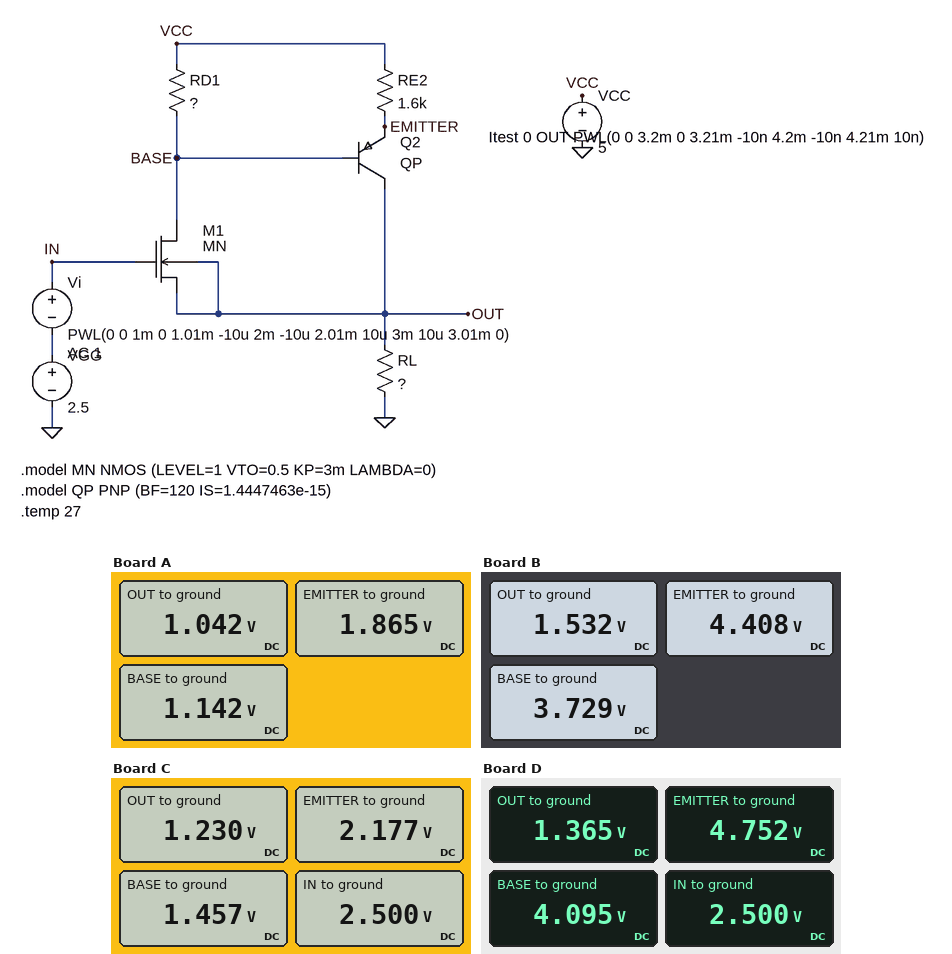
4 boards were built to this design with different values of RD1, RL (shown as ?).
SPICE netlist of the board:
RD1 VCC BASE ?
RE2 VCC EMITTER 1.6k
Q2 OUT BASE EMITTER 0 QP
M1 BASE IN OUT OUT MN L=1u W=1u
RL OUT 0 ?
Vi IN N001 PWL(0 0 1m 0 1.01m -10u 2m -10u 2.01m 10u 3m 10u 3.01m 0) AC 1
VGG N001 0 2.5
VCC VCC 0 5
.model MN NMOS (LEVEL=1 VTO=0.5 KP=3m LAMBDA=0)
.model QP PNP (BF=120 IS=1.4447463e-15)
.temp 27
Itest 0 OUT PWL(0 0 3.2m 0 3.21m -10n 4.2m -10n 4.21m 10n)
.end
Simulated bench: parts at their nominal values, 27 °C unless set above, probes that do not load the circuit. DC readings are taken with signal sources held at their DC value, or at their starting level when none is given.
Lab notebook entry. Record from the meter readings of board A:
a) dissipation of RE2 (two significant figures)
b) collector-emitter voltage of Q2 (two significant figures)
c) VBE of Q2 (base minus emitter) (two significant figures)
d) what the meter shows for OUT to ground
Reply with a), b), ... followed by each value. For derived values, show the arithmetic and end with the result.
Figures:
a) (5 V - 1.865 V)^2 / 1.6 kΩ = 6.1 mW
b) 1.042 V - 1.865 V = -820 mV
c) 1.142 V - 1.865 V = -720 mV
d) 1.042 V
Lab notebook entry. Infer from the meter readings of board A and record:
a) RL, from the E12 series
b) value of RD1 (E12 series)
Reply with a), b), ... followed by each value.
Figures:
a) 470 Ω
b) 15 kΩ
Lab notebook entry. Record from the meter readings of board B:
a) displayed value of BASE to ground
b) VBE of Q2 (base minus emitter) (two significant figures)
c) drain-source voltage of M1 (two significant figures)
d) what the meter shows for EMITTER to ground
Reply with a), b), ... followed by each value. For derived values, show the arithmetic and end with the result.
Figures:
a) 3.729 V
b) 3.729 V - 4.408 V = -680 mV
c) 3.729 V - 1.532 V = 2.2 V
d) 4.408 V
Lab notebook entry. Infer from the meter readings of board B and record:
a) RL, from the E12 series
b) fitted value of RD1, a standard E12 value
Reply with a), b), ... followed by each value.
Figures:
a) 2.2 kΩ
b) 3.9 kΩ
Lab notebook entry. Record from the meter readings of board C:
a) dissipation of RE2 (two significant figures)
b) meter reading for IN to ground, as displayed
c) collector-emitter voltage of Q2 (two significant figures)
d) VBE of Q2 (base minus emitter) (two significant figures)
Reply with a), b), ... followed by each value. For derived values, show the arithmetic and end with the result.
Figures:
a) (5 V - 2.177 V)^2 / 1.6 kΩ = 5.0 mW
b) 2.500 V
c) 1.23 V - 2.177 V = -950 mV
d) 1.457 V - 2.177 V = -720 mV
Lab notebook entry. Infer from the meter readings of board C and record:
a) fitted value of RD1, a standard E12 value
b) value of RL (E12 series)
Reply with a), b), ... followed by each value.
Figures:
a) 8.2 kΩ
b) 560 Ω
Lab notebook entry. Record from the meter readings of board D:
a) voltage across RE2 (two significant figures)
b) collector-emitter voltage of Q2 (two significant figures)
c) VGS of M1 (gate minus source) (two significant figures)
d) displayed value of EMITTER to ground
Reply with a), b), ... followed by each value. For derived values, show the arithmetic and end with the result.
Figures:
a) 5 V - 4.752 V = 250 mV
b) 1.365 V - 4.752 V = -3.4 V
c) 2.5 V - 1.365 V = 1.1 V
d) 4.752 V
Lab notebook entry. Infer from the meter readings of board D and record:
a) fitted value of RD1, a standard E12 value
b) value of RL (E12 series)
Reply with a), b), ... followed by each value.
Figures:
a) 1.5 kΩ
b) 1.8 kΩ
